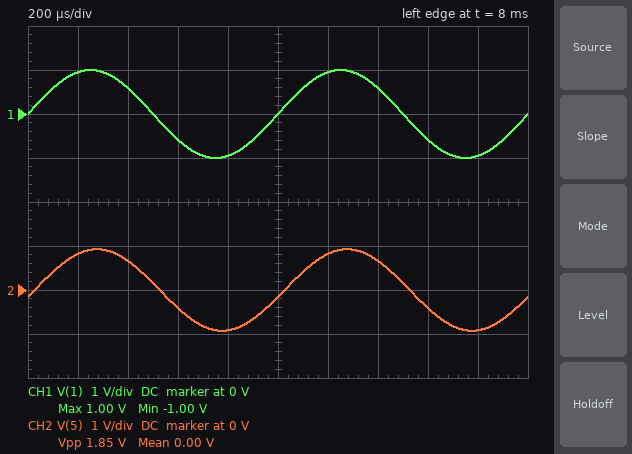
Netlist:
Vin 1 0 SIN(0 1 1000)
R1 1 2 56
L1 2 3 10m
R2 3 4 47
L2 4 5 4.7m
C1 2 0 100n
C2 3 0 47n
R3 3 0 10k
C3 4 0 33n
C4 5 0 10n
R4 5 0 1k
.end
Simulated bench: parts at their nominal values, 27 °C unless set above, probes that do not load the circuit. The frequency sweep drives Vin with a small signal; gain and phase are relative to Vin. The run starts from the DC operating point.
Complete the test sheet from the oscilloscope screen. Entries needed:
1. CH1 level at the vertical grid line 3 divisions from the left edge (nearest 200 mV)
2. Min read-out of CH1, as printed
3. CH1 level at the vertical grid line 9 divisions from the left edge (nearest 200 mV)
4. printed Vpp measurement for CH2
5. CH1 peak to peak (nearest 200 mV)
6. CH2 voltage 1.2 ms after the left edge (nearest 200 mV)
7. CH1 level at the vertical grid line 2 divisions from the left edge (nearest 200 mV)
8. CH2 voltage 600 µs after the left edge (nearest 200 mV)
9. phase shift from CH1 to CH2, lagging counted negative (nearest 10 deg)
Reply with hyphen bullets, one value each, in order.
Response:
- -600 mV
- -1.00 V
- -1.0 V
- 1.85 V
- 2.0 V
- 800 mV
- 600 mV
- -400 mV
- -10 deg
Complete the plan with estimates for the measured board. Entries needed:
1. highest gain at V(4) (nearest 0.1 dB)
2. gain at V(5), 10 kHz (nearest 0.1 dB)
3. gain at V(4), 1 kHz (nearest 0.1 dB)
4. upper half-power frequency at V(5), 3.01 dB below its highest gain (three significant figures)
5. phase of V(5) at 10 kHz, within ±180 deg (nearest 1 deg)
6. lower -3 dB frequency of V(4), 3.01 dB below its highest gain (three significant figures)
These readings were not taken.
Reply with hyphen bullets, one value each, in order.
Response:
- 4.4 dB
- -7.2 dB
- -0.7 dB
- 6.81 kHz
- 166 deg
- 3.13 kHz
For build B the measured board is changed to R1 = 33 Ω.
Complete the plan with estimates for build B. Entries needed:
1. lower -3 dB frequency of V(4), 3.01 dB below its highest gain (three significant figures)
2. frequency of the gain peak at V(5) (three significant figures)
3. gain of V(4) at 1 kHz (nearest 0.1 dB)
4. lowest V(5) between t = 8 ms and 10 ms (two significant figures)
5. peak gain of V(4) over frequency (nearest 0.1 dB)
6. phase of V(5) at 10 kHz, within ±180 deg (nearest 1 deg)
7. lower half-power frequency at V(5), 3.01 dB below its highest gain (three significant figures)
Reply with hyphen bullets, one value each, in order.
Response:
- 3.47 kHz
- 5.29 kHz
- -0.5 dB
- -950 mV
- 5.5 dB
- 171 deg
- 3.57 kHz
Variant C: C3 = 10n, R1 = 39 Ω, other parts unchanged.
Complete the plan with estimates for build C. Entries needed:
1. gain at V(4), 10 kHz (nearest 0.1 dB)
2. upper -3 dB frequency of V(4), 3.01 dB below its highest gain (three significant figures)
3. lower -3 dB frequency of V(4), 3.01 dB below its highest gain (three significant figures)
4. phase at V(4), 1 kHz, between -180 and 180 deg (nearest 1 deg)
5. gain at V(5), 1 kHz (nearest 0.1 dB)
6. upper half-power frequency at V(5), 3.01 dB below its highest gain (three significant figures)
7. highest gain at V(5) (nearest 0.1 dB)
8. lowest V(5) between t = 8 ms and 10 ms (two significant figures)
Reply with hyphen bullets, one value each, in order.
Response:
- -5.0 dB
- 7.68 kHz
- 3.59 kHz
- -6 deg
- -0.6 dB
- 7.78 kHz
- 5.0 dB
- -940 mV
